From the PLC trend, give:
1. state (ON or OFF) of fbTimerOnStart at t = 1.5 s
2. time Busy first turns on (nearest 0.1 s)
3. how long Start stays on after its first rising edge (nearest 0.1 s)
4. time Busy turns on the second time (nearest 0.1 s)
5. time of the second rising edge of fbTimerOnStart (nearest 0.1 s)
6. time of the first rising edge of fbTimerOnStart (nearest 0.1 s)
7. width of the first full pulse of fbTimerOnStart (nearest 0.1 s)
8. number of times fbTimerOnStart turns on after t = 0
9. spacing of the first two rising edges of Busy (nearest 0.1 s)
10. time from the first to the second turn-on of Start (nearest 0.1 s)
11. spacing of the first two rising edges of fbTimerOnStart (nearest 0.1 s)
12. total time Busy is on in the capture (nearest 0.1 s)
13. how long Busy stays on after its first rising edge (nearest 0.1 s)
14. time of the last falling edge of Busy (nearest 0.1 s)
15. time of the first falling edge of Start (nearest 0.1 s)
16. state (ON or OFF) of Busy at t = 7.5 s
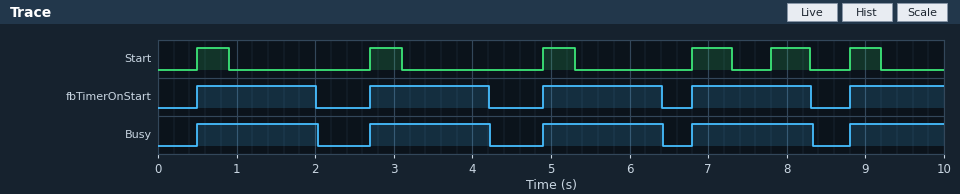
ON
0.5 s
0.4 s
2.7 s
2.7 s
0.5 s
1.5 s
5
2.2 s
2.2 s
2.2 s
7.3 s
1.5 s
8.3 s
0.9 s
ON
